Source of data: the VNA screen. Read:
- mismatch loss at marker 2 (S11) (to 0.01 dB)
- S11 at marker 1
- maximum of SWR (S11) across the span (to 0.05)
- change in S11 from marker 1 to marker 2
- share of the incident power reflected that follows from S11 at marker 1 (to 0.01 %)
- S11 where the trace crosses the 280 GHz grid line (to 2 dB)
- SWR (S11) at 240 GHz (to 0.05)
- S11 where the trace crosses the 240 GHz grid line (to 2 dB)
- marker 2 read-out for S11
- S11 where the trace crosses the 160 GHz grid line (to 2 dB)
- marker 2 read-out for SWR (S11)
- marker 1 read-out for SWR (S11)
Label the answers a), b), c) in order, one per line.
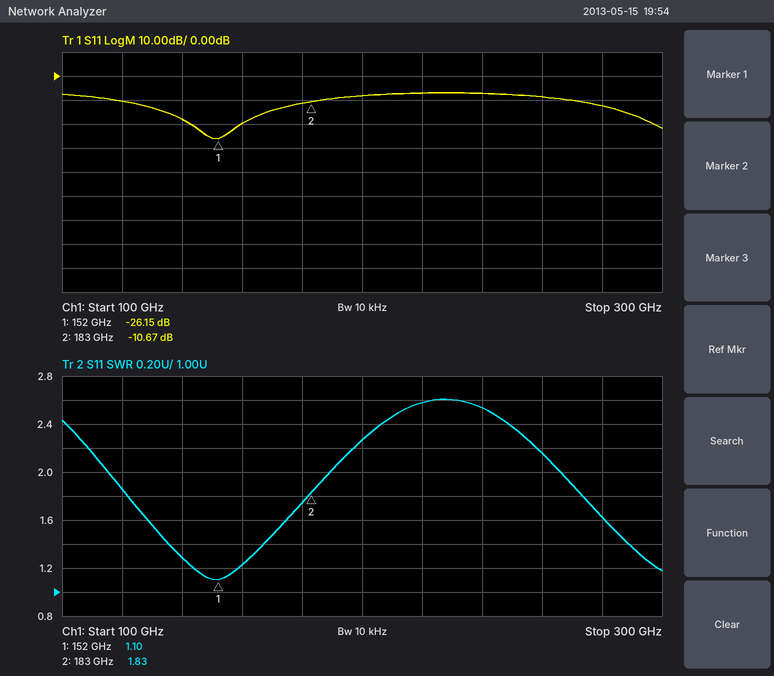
a) 0.39 dB
b) -26.15 dB
c) 2.60
d) 15.48 dB
e) 0.24 %
f) -12 dB
g) 2.55
h) -8 dB
i) -10.67 dB
j) -20 dB
k) 1.83
l) 1.10
